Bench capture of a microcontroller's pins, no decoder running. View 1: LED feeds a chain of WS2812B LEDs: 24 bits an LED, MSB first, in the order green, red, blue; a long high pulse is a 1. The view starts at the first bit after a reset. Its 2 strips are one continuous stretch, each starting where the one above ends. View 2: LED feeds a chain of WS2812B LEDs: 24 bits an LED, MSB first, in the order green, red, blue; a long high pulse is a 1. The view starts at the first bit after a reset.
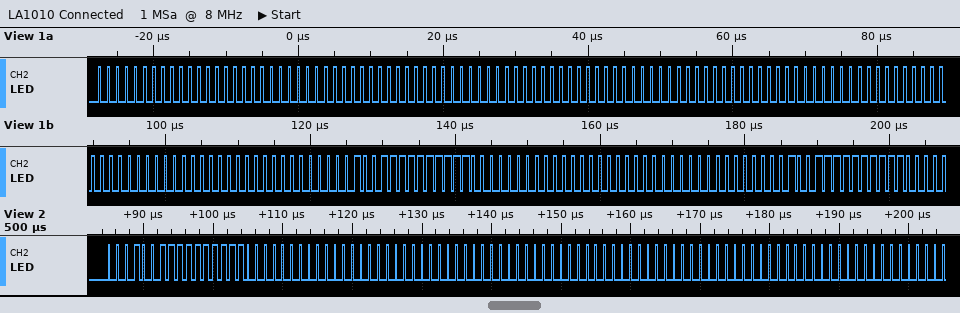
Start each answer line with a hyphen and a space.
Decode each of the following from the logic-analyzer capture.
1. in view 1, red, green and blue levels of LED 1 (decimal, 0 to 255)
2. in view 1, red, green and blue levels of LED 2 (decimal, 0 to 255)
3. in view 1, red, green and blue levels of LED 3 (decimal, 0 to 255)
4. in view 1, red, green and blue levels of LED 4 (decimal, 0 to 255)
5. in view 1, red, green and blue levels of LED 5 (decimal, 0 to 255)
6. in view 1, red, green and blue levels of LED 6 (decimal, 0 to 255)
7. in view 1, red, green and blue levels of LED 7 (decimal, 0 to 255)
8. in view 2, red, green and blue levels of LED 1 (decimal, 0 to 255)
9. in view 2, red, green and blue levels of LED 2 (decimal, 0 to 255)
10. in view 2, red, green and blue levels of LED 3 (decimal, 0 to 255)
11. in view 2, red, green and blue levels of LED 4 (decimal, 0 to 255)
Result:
- 0, 0, 0
- 0, 0, 0
- 0, 0, 0
- 0, 0, 0
- 0, 0, 0
- 255, 19, 0
- 0, 0, 0
- 255, 19, 0
- 0, 0, 0
- 0, 0, 0
- 0, 0, 0
